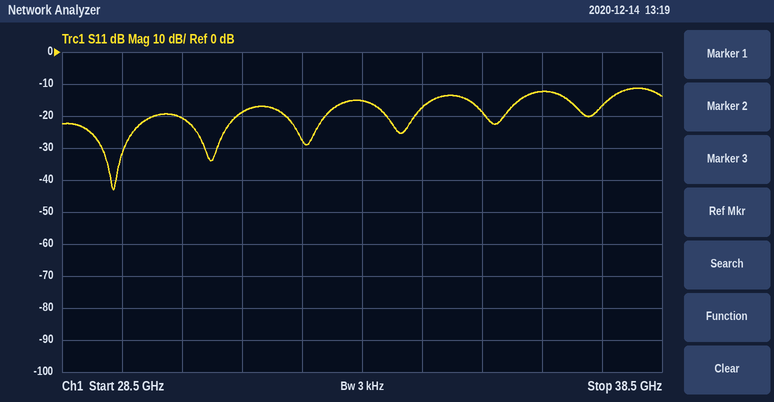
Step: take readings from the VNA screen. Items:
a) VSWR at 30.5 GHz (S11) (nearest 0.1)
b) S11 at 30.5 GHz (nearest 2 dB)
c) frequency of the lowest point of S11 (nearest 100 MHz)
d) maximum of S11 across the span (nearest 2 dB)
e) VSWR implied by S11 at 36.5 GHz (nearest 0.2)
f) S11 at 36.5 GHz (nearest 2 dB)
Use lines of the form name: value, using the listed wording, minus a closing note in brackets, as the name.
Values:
VSWR at 30.5 GHz (S11): 1.2
S11 at 30.5 GHz: -20 dB
frequency of the lowest point of S11: 29.4 GHz
maximum of S11 across the span: -12 dB
VSWR implied by S11 at 36.5 GHz: 1.6
S11 at 36.5 GHz: -12 dB
